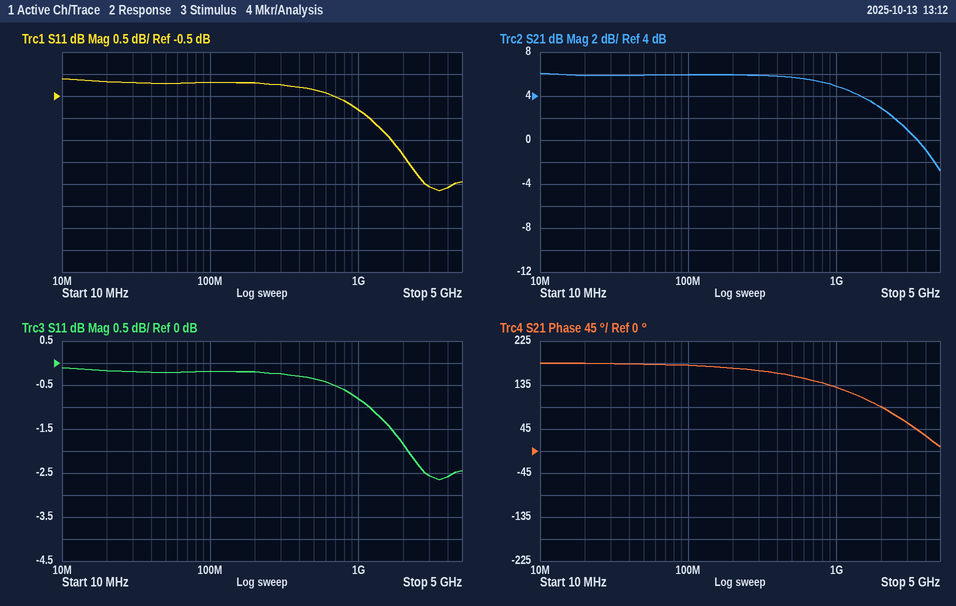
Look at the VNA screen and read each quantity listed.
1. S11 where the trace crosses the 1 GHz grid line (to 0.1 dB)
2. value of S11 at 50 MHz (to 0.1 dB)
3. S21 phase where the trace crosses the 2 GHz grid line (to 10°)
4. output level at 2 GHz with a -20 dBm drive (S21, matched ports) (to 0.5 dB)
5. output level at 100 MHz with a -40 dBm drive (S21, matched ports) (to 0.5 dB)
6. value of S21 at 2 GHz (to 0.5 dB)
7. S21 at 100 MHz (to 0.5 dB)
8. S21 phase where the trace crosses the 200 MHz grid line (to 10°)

-0.8 dB
-0.2 dB
90°
-17.0 dBm
-34.0 dBm
3.0 dB
6.0 dB
170°
